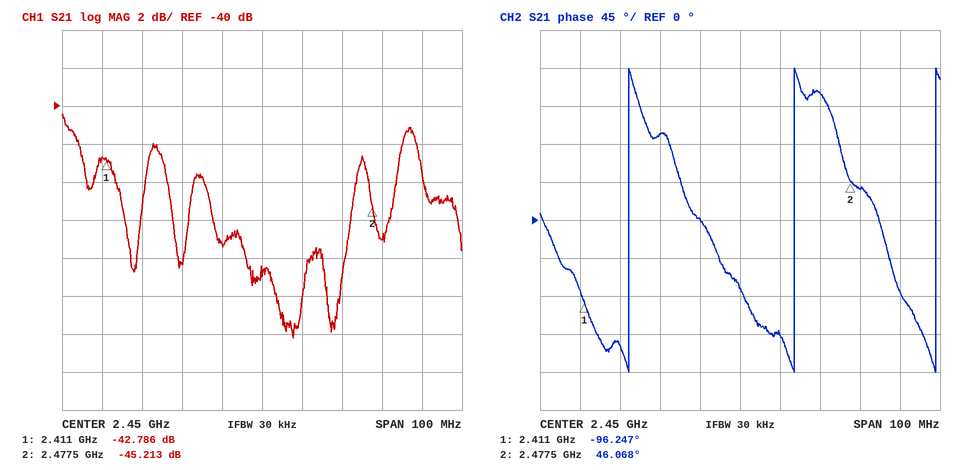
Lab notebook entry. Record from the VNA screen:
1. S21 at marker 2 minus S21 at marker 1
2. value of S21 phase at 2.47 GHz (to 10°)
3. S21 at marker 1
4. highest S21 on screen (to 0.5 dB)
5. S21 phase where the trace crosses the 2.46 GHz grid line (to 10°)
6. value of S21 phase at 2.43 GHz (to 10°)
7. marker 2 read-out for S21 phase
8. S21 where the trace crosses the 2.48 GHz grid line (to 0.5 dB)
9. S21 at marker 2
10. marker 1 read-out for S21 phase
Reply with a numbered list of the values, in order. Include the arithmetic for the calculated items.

1. -45.213 − (-42.786) = -2.427 dB
2. 150°
3. -42.786 dB
4. -40.5 dB
5. -140°
6. 100°
7. 46.068°
8. -47.0 dB
9. -45.213 dB
10. -96.247°
